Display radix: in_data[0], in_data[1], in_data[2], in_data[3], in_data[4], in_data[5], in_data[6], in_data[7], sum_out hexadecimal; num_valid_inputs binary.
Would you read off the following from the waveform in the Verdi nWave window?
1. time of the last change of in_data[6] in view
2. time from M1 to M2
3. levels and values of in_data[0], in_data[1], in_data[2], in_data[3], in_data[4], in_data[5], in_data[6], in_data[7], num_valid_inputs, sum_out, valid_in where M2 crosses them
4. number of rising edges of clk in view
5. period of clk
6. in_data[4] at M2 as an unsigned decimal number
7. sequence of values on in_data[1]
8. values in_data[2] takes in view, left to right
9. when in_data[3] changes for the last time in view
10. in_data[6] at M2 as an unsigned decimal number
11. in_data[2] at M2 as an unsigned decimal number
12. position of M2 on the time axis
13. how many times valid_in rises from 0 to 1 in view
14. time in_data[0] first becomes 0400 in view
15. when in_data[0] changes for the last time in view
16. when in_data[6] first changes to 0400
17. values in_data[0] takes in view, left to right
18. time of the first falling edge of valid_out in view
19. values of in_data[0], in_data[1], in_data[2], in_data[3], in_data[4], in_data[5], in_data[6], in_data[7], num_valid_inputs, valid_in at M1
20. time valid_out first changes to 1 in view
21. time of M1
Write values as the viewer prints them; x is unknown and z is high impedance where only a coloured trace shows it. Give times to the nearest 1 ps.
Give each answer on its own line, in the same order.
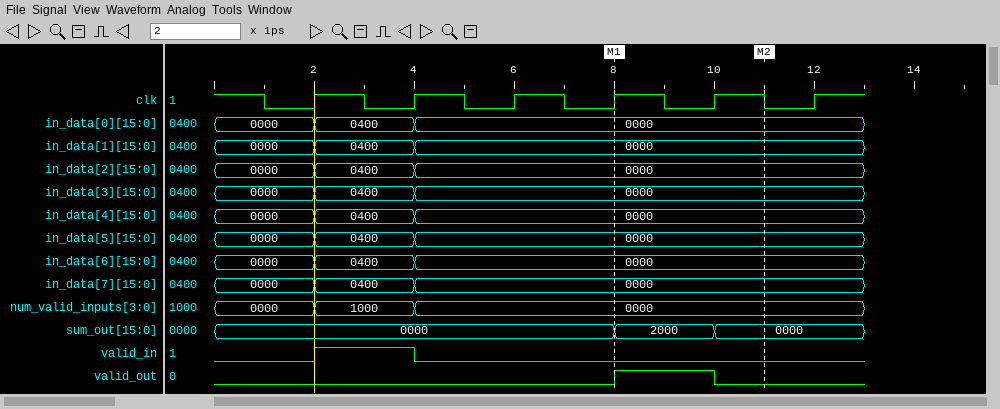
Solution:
4 ps
3 ps
in_data[0]=0000, in_data[1]=0000, in_data[2]=0000, in_data[3]=0000, in_data[4]=0000, in_data[5]=0000, in_data[6]=0000, in_data[7]=0000, num_valid_inputs=0000, sum_out=0000, valid_in=0
6
2 ps
0
0000, 0400, 0000
0000, 0400, 0000
4 ps
0
0
11 ps
1
2 ps
4 ps
2 ps
0000, 0400, 0000
10 ps
in_data[0]=0000, in_data[1]=0000, in_data[2]=0000, in_data[3]=0000, in_data[4]=0000, in_data[5]=0000, in_data[6]=0000, in_data[7]=0000, num_valid_inputs=0000, valid_in=0
8 ps
8 ps
